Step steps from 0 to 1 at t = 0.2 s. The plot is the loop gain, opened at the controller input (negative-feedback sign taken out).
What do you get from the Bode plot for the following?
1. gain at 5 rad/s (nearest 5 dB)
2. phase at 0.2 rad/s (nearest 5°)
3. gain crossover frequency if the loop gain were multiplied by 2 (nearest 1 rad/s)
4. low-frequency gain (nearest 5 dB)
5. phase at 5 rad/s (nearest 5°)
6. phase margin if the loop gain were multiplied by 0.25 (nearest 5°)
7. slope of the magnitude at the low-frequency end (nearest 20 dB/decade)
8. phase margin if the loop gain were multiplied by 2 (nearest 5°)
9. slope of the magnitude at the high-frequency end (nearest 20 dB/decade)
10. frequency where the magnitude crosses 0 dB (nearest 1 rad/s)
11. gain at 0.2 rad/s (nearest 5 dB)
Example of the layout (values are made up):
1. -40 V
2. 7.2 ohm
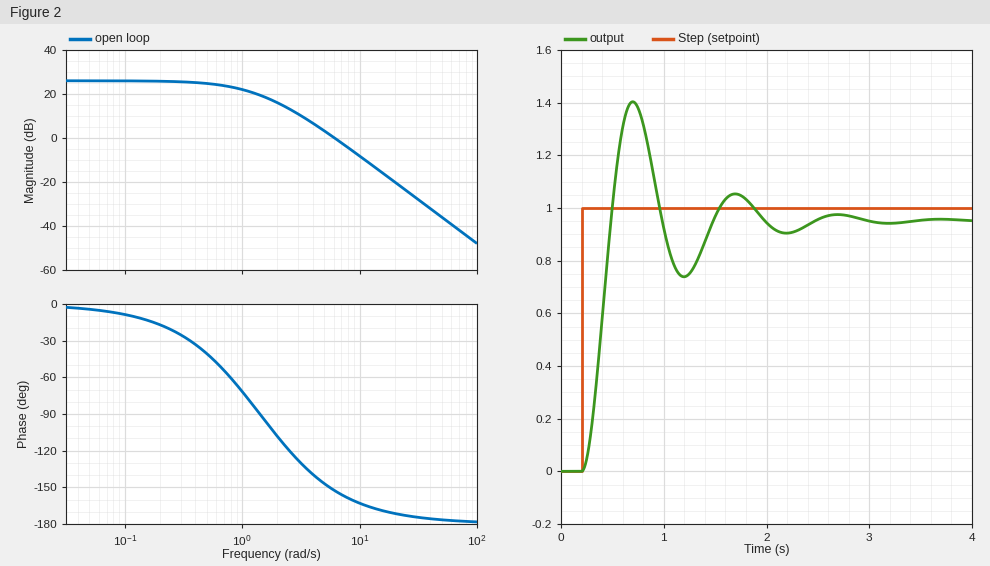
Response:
1. 5 dB
2. -15°
3. 9 rad/s
4. 25 dB
5. -145°
6. 55°
7. 0 dB/decade
8. 20°
9. -40 dB/decade
10. 6 rad/s
11. 25 dB
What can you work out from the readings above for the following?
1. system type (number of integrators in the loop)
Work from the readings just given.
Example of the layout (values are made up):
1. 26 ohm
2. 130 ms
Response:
1. 0
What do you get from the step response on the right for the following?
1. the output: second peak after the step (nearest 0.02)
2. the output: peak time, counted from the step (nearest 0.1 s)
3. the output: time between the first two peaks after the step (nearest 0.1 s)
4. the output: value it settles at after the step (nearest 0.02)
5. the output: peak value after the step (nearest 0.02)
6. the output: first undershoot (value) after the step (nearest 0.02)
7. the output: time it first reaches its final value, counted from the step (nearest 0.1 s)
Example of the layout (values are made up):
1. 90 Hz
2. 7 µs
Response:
1. 1.06
2. 0.5 s
3. 1.0 s
4. 0.96
5. 1.40
6. 0.74
7. 0.3 s
